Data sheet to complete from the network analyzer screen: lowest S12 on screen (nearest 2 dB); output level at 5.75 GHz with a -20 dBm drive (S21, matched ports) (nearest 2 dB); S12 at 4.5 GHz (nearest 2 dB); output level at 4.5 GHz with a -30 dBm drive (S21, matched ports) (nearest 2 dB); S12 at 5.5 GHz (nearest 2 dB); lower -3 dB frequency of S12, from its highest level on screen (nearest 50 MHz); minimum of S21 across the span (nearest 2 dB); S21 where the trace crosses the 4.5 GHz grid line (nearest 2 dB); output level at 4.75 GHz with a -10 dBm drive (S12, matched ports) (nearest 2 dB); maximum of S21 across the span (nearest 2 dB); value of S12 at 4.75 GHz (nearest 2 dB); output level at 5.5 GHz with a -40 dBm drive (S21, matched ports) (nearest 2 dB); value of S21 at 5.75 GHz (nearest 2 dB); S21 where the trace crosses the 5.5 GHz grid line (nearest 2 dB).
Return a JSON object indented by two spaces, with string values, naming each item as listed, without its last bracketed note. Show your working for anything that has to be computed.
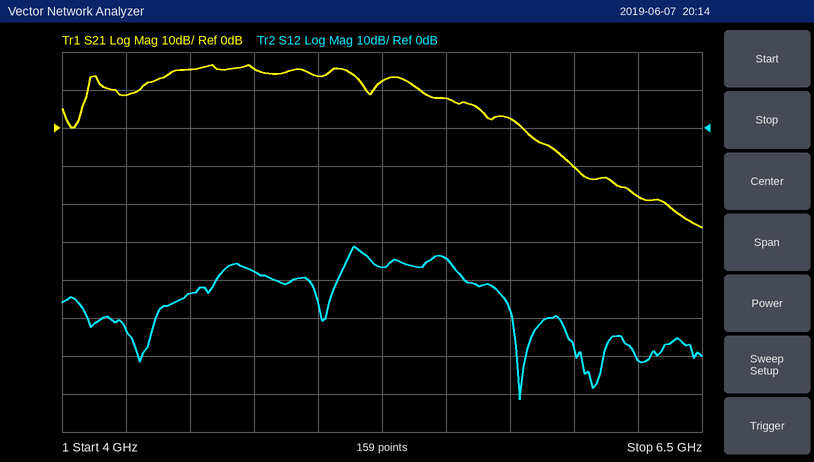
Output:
{
  "lowest S12 on screen": "-72 dB",
  "output level at 5.75 GHz with a -20 dBm drive (S21, matched ports)": "-20 dBm + (2 dB) = -18 dBm",
  "S12 at 4.5 GHz": "-44 dB",
  "output level at 4.5 GHz with a -30 dBm drive (S21, matched ports)": "-30 dBm + (16 dB) = -14 dBm",
  "S12 at 5.5 GHz": "-34 dB",
  "lower -3 dB frequency of S12, from its highest level on screen": "5.10 GHz",
  "minimum of S21 across the span": "-26 dB",
  "S21 where the trace crosses the 4.5 GHz grid line": "16 dB",
  "output level at 4.75 GHz with a -10 dBm drive (S12, matched ports)": "-10 dBm + (-38 dB) = -48 dBm",
  "maximum of S21 across the span": "16 dB",
  "value of S12 at 4.75 GHz": "-38 dB",
  "output level at 5.5 GHz with a -40 dBm drive (S21, matched ports)": "-40 dBm + (8 dB) = -32 dBm",
  "value of S21 at 5.75 GHz": "2 dB",
  "S21 where the trace crosses the 5.5 GHz grid line": "8 dB"
}
